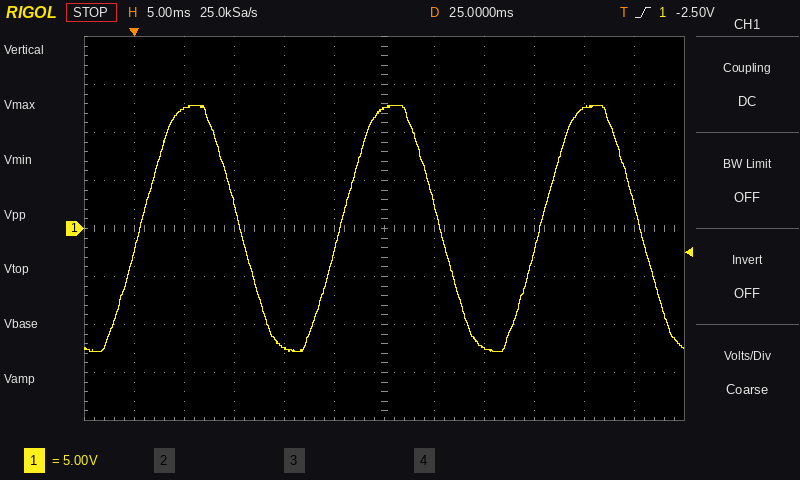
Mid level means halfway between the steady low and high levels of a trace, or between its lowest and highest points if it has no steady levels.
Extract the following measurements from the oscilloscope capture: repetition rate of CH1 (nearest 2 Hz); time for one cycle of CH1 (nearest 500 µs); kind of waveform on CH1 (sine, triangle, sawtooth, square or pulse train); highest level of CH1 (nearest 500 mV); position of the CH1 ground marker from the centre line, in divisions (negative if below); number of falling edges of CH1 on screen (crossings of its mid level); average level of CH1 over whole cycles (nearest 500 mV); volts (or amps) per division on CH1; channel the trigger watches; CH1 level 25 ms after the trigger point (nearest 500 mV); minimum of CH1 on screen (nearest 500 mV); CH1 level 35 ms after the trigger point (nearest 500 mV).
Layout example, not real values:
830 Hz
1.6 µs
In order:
50 Hz
20.0 ms
sine
13.0 V
0.0 div
3
0.0 V
5 V
CH1
12.5 V
-13.0 V
-12.5 V
